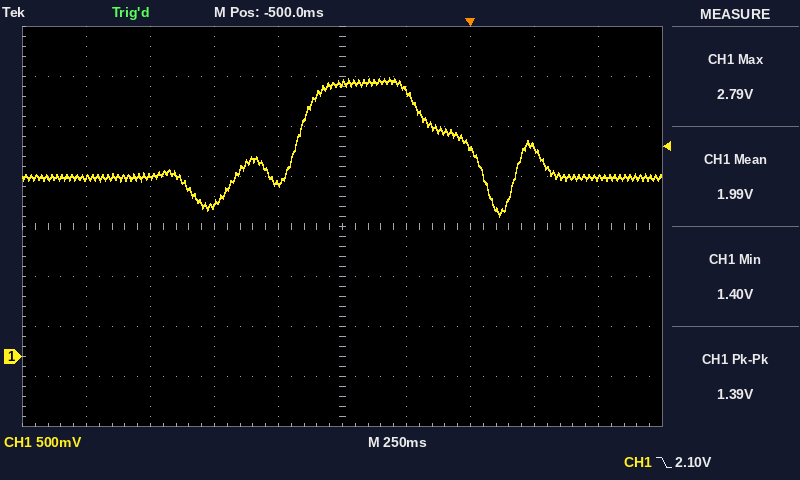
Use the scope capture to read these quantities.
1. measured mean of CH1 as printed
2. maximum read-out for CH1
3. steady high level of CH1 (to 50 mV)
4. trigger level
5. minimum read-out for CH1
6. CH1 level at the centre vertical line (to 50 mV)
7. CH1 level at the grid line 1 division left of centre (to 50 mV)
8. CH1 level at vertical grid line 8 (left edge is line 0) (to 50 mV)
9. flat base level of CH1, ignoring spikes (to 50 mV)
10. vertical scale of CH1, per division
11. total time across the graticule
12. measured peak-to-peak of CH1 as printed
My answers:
1.99 V
2.79 V
2.75 V
2.10 V
1.40 V
2.75 V
1.75 V
2.10 V
1.80 V
500 mV
2.5 s
1.39 V
